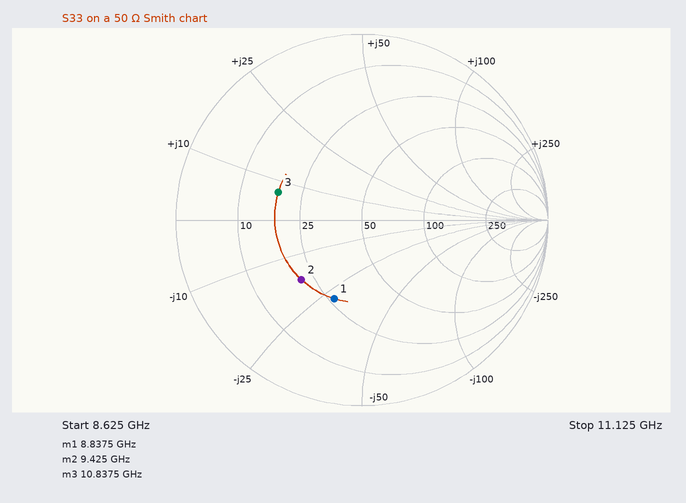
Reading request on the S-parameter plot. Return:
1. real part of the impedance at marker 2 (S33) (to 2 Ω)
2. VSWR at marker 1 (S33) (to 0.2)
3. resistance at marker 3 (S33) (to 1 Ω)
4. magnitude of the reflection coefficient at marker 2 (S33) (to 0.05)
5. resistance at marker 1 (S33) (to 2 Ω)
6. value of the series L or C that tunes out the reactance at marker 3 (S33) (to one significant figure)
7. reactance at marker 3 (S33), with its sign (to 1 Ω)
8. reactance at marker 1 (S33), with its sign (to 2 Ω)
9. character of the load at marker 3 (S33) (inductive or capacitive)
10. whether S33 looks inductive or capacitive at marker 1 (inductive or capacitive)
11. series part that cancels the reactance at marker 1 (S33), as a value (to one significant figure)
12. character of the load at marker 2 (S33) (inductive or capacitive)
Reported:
22 Ω
2.6
18 Ω
0.45
26 Ω
2 pF
+7 Ω
-28 Ω
inductive
capacitive
500 pH
capacitive
